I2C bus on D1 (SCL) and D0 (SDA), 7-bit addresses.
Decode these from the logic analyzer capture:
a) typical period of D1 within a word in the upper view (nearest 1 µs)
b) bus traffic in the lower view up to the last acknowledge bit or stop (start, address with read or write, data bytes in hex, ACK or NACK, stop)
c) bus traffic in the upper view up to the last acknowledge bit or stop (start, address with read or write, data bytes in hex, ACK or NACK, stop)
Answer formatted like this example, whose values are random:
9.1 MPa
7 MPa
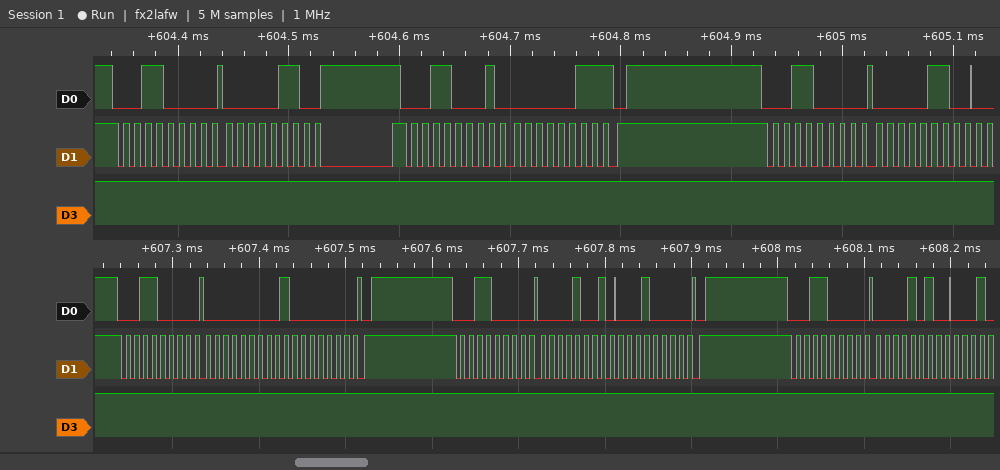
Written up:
10 µs
start, address 18 write ACK, 00 ACK, 80 ACK, stop, start, address 18 write ACK, 09 ACK, 10 ACK, stop, start, address 18 write ACK, 0A ACK
start, address 18 write ACK, 06 ACK, repeated start, address 18 read ACK, 03 NACK, stop, start, address 18 write ACK, 06 ACK
